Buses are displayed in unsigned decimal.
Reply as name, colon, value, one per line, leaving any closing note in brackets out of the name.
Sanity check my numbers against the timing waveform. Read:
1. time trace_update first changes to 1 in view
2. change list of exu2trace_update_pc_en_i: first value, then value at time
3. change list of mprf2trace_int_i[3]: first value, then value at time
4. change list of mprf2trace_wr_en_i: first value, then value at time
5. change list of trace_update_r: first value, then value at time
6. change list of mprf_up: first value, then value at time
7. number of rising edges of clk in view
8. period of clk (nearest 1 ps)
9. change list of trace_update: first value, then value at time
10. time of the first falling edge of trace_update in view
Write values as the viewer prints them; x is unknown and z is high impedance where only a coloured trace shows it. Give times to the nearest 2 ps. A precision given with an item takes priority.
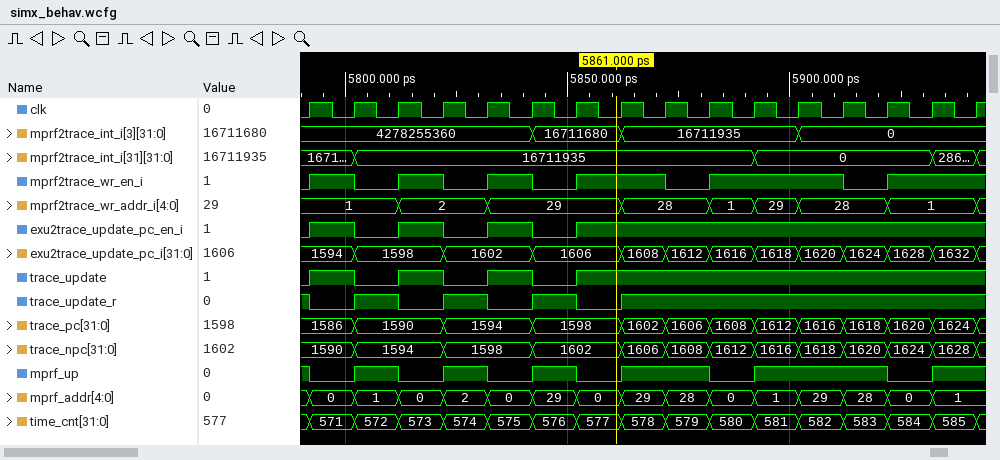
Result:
time trace_update first changes to 1 in view: 5792 ps
change list of exu2trace_update_pc_en_i: first value, then value at time: 0, 1 at 5792 ps, 0 at 5802 ps, 1 at 5812 ps, 0 at 5822 ps, 1 at 5832 ps, 0 at 5842 ps, 1 at 5852 ps
change list of mprf2trace_int_i[3]: first value, then value at time: 4278255360, 16711680 at 5842 ps, 16711935 at 5862 ps, 0 at 5902 ps
change list of mprf2trace_wr_en_i: first value, then value at time: 0, 1 at 5792 ps, 0 at 5802 ps, 1 at 5812 ps, 0 at 5822 ps, 1 at 5832 ps, 0 at 5842 ps, 1 at 5852 ps, 0 at 5872 ps, 1 at 5882 ps, 0 at 5912 ps, 1 at 5922 ps
change list of trace_update_r: first value, then value at time: 1, 0 at 5792 ps, 1 at 5802 ps, 0 at 5812 ps, 1 at 5822 ps, 0 at 5832 ps, 1 at 5842 ps, 0 at 5852 ps, 1 at 5862 ps
change list of mprf_up: first value, then value at time: 1, 0 at 5792 ps, 1 at 5802 ps, 0 at 5812 ps, 1 at 5822 ps, 0 at 5832 ps, 1 at 5842 ps, 0 at 5852 ps, 1 at 5862 ps, 0 at 5882 ps, 1 at 5892 ps, 0 at 5922 ps, 1 at 5932 ps
number of rising edges of clk in view: 16
period of clk: 10 ps
change list of trace_update: first value, then value at time: 0, 1 at 5792 ps, 0 at 5802 ps, 1 at 5812 ps, 0 at 5822 ps, 1 at 5832 ps, 0 at 5842 ps, 1 at 5852 ps
time of the first falling edge of trace_update in view: 5802 ps
